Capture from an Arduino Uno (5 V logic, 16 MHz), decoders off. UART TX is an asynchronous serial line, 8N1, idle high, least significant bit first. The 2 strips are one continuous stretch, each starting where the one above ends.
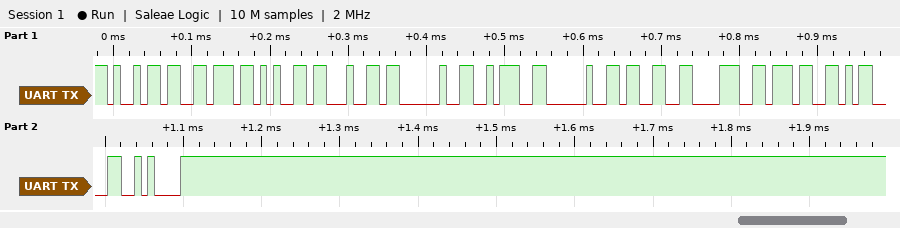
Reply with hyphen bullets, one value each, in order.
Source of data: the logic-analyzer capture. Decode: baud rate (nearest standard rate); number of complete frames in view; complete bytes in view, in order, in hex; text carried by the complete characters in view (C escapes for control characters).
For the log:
- 115200 baud
- 12
- 0x69 0x76 0x65 0x64 0x20 0x3A 0x20 0x33 0x38 0x37 0x0D 0x0A
- "ived : 387\r\n"
